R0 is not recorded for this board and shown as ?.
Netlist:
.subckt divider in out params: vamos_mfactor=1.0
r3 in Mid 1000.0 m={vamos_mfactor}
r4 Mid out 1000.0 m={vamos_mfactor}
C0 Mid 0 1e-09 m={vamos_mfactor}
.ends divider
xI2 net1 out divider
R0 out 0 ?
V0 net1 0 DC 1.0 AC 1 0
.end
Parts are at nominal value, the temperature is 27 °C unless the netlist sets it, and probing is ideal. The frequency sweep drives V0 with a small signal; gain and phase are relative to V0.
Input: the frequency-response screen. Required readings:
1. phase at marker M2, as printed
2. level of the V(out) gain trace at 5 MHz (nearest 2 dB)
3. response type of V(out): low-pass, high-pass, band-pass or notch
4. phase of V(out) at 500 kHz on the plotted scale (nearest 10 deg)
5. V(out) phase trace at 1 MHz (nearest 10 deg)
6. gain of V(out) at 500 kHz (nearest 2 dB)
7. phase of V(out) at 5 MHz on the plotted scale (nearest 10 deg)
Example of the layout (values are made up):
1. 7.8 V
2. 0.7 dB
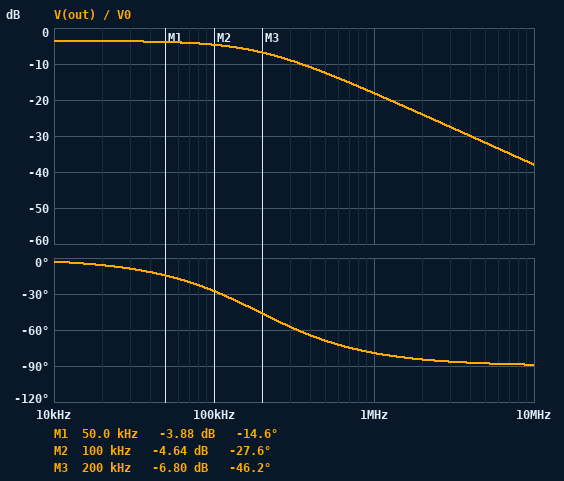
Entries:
1. -27.6 deg
2. -32 dB
3. low-pass
4. -70 deg
5. -80 deg
6. -12 dB
7. -90 deg
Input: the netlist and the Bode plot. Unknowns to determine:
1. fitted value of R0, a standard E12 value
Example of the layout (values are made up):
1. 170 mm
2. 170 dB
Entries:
1. 3.9 kΩ
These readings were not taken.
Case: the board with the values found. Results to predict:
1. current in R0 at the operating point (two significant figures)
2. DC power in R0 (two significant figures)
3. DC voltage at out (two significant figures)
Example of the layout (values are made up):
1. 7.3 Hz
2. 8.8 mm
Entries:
1. 170 µA
2. 110 µW
3. 660 mV
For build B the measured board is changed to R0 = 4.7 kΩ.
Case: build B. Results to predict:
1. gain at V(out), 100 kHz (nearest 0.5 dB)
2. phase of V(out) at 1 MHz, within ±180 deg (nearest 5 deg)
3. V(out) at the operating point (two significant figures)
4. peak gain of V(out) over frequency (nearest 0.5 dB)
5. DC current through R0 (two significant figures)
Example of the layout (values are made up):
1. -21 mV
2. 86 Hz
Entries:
1. -4.0 dB
2. -80 deg
3. 700 mV
4. -3.0 dB
5. 150 µA
